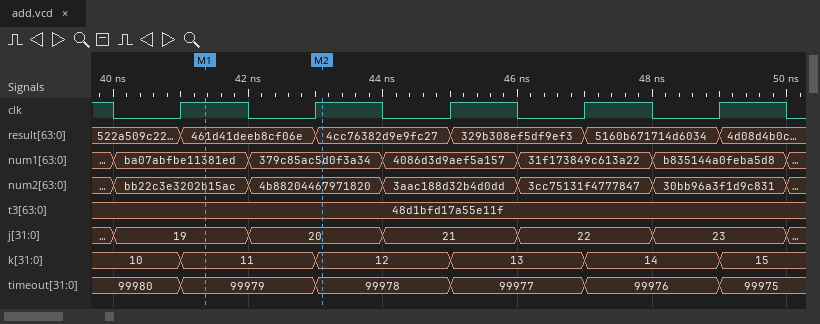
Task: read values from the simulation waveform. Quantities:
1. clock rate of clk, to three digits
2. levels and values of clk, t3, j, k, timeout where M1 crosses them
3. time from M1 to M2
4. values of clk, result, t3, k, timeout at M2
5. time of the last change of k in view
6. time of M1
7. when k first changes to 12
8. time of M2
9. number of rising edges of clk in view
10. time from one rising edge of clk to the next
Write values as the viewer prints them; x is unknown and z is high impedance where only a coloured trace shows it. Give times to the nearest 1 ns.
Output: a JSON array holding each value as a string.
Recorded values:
["500 MHz", "clk=1, t3=48d1bfd17a55e11f, j=19, k=11, timeout=99979", "2 ns", "clk=1, result=4cc76382d9e9fc27, t3=48d1bfd17a55e11f, k=12, timeout=99978", "49 ns", "41 ns", "43 ns", "43 ns", "5", "2 ns"]
